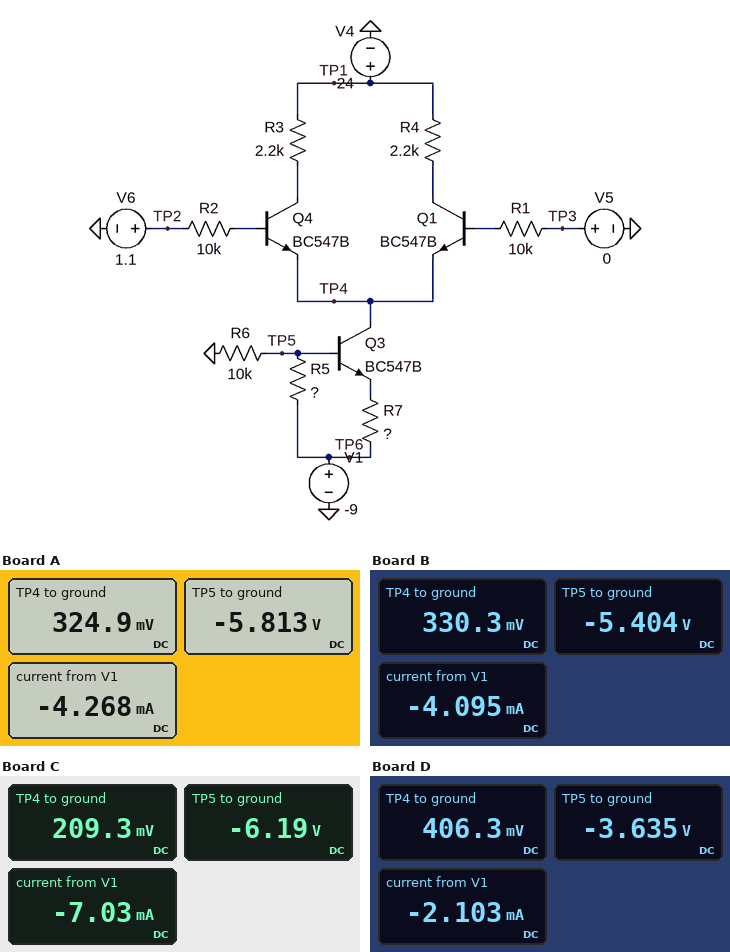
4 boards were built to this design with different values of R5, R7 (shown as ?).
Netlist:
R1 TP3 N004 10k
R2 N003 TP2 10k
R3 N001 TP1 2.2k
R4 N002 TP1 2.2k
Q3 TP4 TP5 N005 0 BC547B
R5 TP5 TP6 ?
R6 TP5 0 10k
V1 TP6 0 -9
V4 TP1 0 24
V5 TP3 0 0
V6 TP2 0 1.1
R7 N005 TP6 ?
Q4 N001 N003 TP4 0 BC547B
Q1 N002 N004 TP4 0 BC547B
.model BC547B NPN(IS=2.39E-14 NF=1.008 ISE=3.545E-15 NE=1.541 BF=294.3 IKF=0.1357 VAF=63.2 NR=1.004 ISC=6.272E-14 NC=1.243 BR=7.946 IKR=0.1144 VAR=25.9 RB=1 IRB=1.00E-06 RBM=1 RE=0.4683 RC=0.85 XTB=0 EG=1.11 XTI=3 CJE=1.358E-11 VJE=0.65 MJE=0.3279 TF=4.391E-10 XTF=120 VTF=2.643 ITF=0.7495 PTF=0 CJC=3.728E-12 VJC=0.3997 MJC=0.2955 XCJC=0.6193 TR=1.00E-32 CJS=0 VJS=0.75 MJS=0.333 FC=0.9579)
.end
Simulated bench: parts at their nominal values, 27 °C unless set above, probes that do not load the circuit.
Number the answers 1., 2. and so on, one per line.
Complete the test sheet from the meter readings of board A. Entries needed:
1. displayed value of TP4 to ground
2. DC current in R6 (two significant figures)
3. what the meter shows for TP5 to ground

1. 324.9 mV
2. 580 µA
3. -5.813 V
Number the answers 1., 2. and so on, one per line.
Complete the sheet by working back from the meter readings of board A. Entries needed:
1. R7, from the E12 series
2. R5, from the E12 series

1. 680 Ω
2. 5.6 kΩ
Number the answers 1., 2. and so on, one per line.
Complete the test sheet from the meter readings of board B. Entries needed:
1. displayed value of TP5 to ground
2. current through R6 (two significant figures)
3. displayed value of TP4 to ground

1. -5.404 V
2. 540 µA
3. 330.3 mV
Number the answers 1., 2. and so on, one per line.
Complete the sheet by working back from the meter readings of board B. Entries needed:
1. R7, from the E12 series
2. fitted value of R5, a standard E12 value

1. 820 Ω
2. 6.8 kΩ
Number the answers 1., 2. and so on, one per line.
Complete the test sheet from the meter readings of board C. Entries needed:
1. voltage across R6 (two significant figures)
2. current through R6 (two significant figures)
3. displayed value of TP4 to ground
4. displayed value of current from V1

1. 6.2 V
2. 620 µA
3. 209.3 mV
4. -7.03 mA
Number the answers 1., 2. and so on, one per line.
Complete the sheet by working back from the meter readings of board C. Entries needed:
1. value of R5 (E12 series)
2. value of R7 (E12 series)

1. 4.7 kΩ
2. 330 Ω
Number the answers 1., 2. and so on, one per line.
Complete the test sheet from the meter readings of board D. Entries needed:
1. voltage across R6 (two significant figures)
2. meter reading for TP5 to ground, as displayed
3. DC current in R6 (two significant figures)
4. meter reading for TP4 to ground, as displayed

1. 3.6 V
2. -3.635 V
3. 360 µA
4. 406.3 mV
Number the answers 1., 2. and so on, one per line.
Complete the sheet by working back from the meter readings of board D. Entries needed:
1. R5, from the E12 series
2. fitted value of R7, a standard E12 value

1. 15 kΩ
2. 2.7 kΩ
